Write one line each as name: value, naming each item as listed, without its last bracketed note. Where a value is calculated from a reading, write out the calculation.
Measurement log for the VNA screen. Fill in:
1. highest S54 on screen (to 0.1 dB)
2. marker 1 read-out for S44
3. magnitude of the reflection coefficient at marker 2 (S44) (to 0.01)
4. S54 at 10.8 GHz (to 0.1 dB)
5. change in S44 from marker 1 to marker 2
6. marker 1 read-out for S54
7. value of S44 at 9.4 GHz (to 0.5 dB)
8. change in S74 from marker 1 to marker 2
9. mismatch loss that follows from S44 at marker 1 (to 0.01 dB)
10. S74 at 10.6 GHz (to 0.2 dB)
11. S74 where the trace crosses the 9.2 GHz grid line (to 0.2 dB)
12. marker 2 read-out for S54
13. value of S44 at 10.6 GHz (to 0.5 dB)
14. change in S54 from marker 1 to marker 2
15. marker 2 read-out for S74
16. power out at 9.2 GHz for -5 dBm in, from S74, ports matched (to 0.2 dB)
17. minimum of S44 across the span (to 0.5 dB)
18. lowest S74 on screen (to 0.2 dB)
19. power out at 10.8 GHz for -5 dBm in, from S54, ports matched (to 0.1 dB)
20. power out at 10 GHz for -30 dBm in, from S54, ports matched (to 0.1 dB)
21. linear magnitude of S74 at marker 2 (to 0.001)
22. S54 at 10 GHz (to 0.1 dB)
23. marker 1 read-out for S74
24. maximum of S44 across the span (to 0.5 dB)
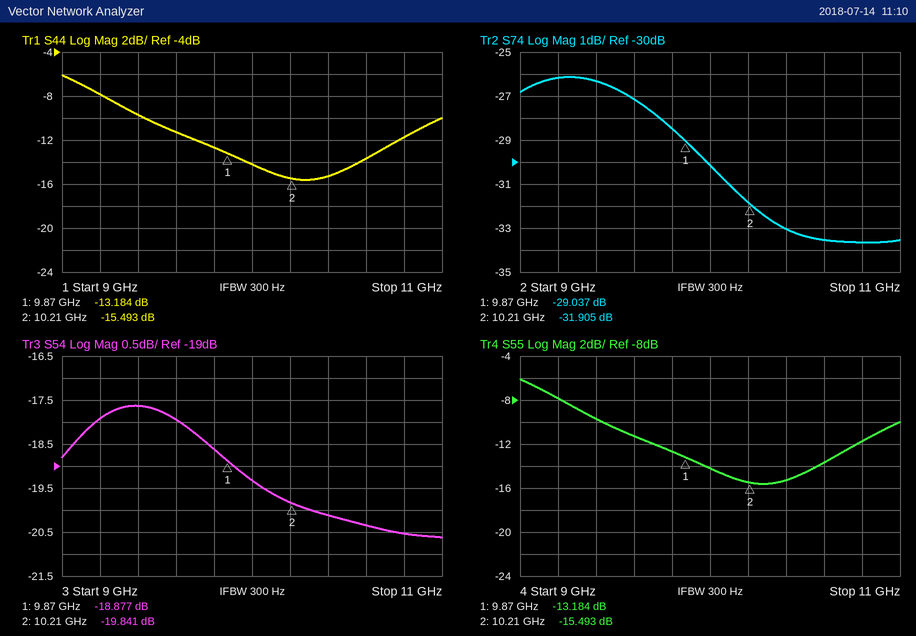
highest S54 on screen: -17.6 dB
marker 1 read-out for S44: -13.184 dB
magnitude of the reflection coefficient at marker 2 (S44): 10^(-15.493/20) ≈ 0.17
S54 at 10.8 GHz: -20.5 dB
change in S44 from marker 1 to marker 2: -15.493 − (-13.184) = -2.309 dB
marker 1 read-out for S54: -18.877 dB
value of S44 at 9.4 GHz: -9.5 dB
change in S74 from marker 1 to marker 2: -31.905 − (-29.037) = -2.868 dB
mismatch loss that follows from S44 at marker 1: −10 log10(1 − 10^(-13.184/10)) ≈ 0.21 dB
S74 at 10.6 GHz: -33.6 dB
S74 where the trace crosses the 9.2 GHz grid line: -26.2 dB
marker 2 read-out for S54: -19.841 dB
value of S44 at 10.6 GHz: -13.5 dB
change in S54 from marker 1 to marker 2: -19.841 − (-18.877) = -0.964 dB
marker 2 read-out for S74: -31.905 dB
power out at 9.2 GHz for -5 dBm in, from S74, ports matched: -5 dBm + (-26.2 dB) = -31.2 dBm
minimum of S44 across the span: -15.5 dB
lowest S74 on screen: -33.6 dB
power out at 10.8 GHz for -5 dBm in, from S54, ports matched: -5 dBm + (-20.5 dB) = -25.5 dBm
power out at 10 GHz for -30 dBm in, from S54, ports matched: -30 dBm + (-19.3 dB) = -49.3 dBm
linear magnitude of S74 at marker 2: 10^(-31.905/20) ≈ 0.025
S54 at 10 GHz: -19.3 dB
marker 1 read-out for S74: -29.037 dB
maximum of S44 across the span: -6.0 dB
